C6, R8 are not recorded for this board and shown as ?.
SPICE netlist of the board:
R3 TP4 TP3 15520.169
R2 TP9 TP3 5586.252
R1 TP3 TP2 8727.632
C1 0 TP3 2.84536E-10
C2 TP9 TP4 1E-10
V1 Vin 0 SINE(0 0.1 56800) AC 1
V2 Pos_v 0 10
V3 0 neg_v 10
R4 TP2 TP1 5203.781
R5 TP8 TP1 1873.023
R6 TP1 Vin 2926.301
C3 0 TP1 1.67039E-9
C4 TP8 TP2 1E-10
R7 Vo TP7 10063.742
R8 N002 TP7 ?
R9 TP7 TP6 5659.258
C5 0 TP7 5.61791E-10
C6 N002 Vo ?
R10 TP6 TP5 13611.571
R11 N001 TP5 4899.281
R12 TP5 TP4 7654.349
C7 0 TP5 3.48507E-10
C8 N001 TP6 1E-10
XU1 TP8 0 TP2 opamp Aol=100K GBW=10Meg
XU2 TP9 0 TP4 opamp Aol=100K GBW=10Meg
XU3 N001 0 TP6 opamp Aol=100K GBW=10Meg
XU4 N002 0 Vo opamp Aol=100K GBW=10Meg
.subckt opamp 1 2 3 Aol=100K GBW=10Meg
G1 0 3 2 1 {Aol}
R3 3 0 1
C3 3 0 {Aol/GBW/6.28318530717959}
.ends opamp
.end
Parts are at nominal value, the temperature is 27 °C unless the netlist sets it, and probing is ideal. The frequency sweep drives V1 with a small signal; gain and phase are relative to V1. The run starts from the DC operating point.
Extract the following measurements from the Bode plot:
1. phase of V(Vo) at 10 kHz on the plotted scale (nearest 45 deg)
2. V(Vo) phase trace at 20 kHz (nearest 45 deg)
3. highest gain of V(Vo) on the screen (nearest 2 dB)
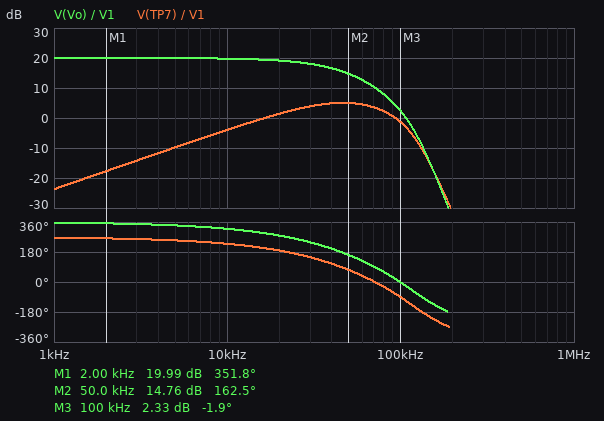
315 deg
270 deg
20 dB
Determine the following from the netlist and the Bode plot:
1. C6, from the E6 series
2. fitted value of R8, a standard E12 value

150 pF
6.8 kΩ
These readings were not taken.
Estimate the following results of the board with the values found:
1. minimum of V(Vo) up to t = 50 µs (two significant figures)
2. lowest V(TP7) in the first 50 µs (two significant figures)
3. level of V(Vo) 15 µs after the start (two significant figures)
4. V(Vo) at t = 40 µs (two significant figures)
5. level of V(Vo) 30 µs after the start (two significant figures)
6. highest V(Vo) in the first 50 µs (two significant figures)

-470 mV
-170 mV
550 mV
-390 mV
240 mV
550 mV
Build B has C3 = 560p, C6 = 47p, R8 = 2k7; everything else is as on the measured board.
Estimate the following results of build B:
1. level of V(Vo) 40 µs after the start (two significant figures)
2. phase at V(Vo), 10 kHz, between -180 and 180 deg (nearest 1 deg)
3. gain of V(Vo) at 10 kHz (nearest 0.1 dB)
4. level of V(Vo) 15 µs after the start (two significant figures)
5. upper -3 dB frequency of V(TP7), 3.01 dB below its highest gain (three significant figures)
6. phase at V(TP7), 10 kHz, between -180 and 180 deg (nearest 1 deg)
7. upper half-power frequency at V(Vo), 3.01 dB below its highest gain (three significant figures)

-570 mV
-28 deg
19.9 dB
330 mV
118 kHz
-118 deg
52.8 kHz
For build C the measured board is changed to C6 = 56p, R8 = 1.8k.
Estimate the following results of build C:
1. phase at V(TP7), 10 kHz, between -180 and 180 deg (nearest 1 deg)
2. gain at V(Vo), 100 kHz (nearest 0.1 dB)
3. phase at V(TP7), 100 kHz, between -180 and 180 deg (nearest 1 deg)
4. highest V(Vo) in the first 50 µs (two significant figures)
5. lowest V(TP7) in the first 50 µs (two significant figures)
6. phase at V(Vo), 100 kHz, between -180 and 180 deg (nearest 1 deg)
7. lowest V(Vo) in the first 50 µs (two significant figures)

-118 deg
12.7 dB
-12 deg
770 mV
-32 mV
77 deg
-760 mV
